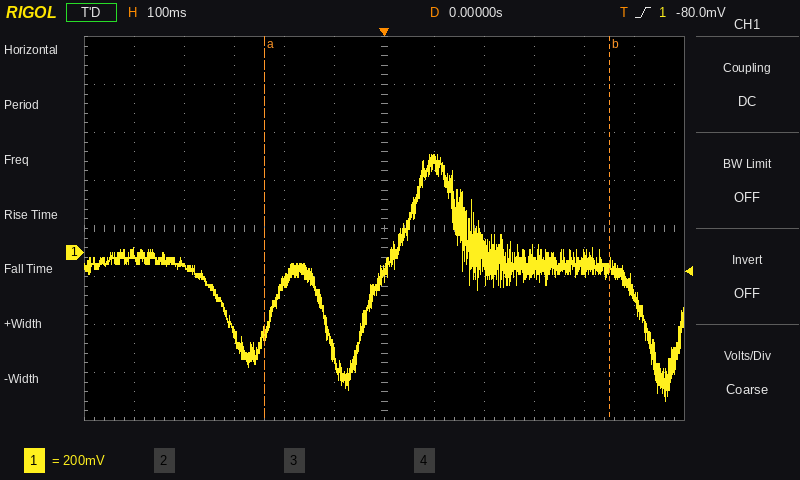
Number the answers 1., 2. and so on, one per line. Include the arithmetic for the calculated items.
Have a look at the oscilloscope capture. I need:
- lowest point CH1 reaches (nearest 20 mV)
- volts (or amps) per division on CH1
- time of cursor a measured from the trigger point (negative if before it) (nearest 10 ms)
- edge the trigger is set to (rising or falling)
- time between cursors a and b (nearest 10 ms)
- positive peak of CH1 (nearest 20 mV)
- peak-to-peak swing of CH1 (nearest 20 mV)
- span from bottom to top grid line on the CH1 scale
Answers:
1. -620 mV
2. 200 mV
3. -240 ms
4. rising
5. 690 ms
6. 400 mV
7. 400 mV − (-620 mV) = 1.02 V
8. 1.6 V
